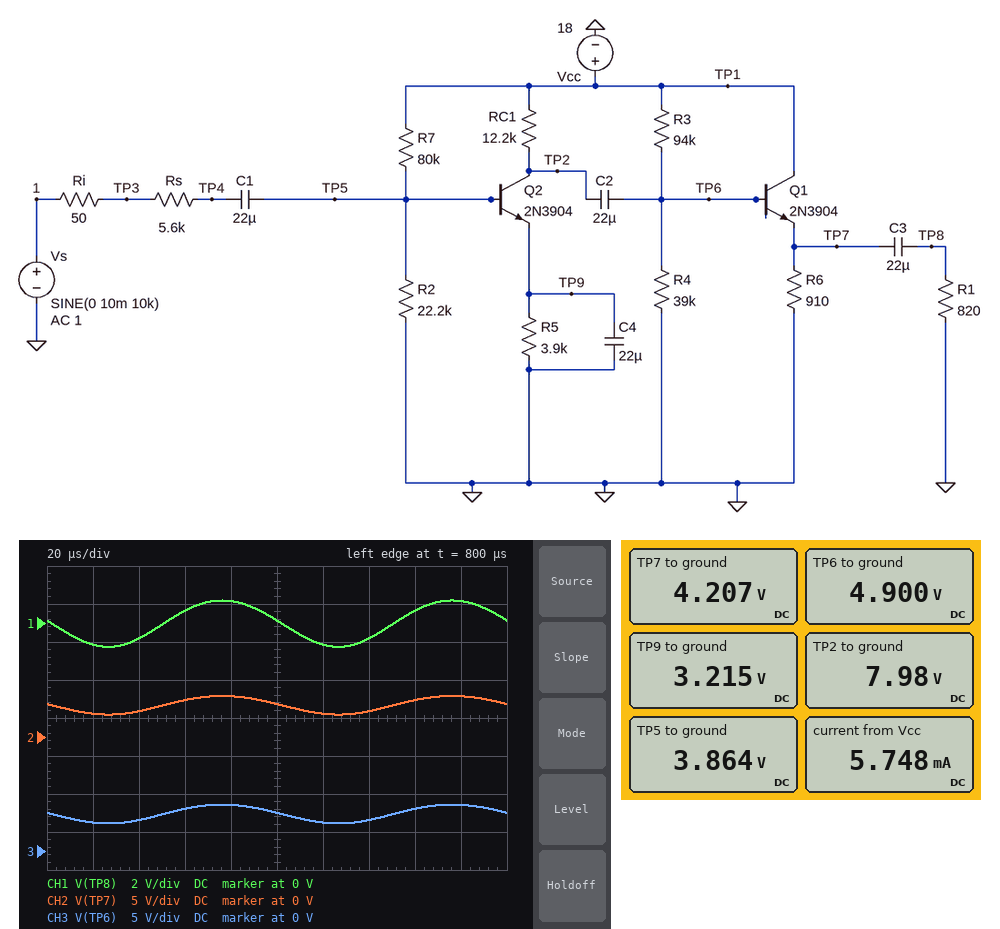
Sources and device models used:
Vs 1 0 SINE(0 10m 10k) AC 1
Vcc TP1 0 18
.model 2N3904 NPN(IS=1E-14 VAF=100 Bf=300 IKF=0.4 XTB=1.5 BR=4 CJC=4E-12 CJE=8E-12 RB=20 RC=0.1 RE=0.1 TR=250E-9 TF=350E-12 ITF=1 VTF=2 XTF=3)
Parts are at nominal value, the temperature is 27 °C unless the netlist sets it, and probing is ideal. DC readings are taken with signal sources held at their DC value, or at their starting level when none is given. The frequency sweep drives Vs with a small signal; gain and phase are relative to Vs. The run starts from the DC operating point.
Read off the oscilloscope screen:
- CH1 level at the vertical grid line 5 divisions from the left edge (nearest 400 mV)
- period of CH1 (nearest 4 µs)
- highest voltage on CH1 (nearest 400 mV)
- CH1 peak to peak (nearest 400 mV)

0 V
100 µs
1.2 V
2.4 V
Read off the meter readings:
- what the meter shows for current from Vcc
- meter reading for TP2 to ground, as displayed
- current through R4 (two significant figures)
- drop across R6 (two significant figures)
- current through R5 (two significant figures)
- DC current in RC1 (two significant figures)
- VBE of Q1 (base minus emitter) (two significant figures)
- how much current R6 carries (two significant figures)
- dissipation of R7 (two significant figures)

5.748 mA
7.98 V
130 µA
4.2 V
820 µA
820 µA
690 mV
4.6 mA
2.5 mW
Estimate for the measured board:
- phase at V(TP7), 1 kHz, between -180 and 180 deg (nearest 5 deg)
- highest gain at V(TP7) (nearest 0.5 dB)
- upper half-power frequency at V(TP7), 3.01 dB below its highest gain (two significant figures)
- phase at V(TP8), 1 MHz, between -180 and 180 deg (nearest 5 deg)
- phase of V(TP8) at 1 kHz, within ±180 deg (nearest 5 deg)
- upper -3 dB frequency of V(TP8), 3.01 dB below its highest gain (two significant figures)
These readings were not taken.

-170 deg
42.0 dB
97 kHz
95 deg
-170 deg
97 kHz
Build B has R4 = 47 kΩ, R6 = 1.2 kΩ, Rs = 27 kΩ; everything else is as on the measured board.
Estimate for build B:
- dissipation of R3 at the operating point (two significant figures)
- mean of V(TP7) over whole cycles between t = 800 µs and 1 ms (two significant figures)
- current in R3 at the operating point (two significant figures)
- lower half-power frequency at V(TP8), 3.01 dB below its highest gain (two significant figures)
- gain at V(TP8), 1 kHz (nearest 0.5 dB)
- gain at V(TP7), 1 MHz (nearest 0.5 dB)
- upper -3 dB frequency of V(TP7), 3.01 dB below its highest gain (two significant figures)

1.6 mW
4.9 V
130 µA
110 Hz
33.0 dB
8.0 dB
55 kHz
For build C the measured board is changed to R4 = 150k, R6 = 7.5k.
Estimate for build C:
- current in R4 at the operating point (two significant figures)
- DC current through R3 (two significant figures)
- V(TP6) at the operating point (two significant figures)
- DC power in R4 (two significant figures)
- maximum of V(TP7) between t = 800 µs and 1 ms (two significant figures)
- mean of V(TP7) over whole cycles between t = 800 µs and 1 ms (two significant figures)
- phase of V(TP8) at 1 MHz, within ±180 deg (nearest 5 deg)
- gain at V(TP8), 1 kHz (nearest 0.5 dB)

72 µA
76 µA
11 V
780 µW
12 V
10 V
95 deg
43.0 dB
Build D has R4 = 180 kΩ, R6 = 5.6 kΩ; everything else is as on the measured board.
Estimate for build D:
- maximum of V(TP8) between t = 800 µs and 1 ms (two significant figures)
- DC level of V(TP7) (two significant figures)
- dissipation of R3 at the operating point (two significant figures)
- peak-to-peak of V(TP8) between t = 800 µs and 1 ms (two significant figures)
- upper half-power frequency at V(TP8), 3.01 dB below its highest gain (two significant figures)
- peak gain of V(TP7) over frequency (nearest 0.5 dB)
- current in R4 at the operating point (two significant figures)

1.4 V
11 V
460 µW
2.8 V
81 kHz
43.5 dB
64 µA
